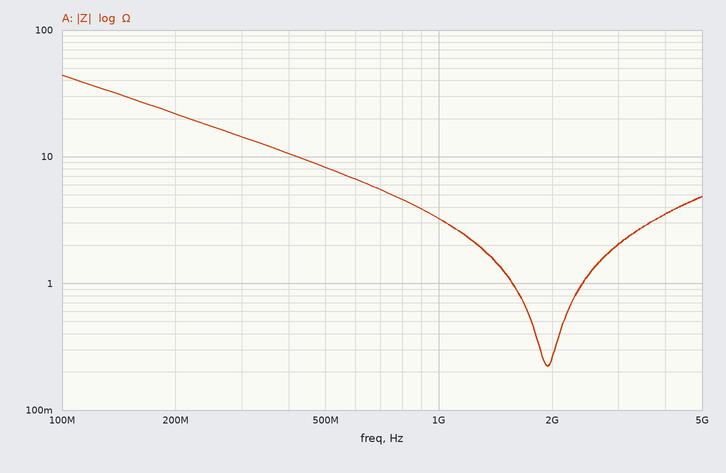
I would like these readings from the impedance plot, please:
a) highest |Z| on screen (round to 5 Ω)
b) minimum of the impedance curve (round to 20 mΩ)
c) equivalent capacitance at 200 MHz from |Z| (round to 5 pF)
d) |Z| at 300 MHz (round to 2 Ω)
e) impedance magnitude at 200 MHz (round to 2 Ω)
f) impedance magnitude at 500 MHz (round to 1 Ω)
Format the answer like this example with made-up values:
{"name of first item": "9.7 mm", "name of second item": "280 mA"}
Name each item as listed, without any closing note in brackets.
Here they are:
{"highest |Z| on screen": "45 Ω", "minimum of the impedance curve": "220 mΩ", "equivalent capacitance at 200 MHz from |Z|": "35 pF", "|Z| at 300 MHz": "14 Ω", "impedance magnitude at 200 MHz": "22 Ω", "impedance magnitude at 500 MHz": "8 Ω"}
